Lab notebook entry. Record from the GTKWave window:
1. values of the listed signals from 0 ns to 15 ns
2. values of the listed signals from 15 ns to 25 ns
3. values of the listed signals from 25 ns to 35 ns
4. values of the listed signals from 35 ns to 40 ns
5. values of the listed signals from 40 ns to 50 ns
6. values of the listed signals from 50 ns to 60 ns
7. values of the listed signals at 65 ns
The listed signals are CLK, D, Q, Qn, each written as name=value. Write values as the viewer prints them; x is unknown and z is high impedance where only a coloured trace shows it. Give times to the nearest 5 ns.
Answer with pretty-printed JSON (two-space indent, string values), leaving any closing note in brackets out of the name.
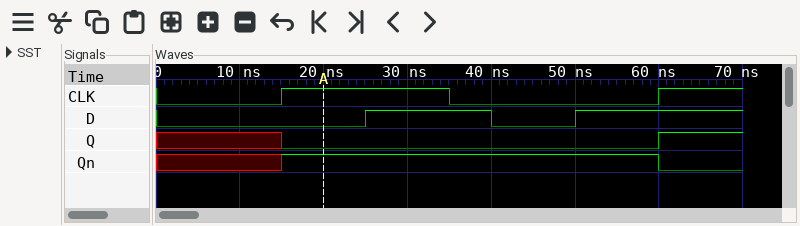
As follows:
{
  "values of the listed signals from 0 ns to 15 ns": "CLK=0, D=0, Q=x, Qn=x",
  "values of the listed signals from 15 ns to 25 ns": "CLK=1, D=0, Q=0, Qn=1",
  "values of the listed signals from 25 ns to 35 ns": "CLK=1, D=1, Q=0, Qn=1",
  "values of the listed signals from 35 ns to 40 ns": "CLK=0, D=1, Q=0, Qn=1",
  "values of the listed signals from 40 ns to 50 ns": "CLK=0, D=0, Q=0, Qn=1",
  "values of the listed signals from 50 ns to 60 ns": "CLK=0, D=1, Q=0, Qn=1",
  "values of the listed signals at 65 ns": "CLK=1, D=1, Q=1, Qn=0"
}
